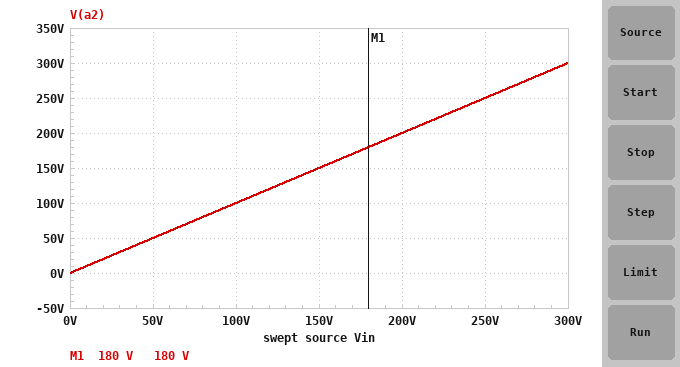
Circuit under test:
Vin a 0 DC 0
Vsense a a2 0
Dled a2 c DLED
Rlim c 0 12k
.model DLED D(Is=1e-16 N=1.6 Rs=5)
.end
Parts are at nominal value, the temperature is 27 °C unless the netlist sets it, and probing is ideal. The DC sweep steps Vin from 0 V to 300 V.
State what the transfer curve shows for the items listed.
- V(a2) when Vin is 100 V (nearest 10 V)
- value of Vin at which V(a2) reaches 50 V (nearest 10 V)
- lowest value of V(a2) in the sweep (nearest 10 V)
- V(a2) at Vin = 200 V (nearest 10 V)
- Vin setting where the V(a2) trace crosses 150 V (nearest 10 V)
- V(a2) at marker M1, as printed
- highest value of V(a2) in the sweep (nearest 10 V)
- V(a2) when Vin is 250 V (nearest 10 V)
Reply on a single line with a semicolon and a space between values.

100 V; 50 V; 0 V; 200 V; 150 V; 180 V; 300 V; 250 V
